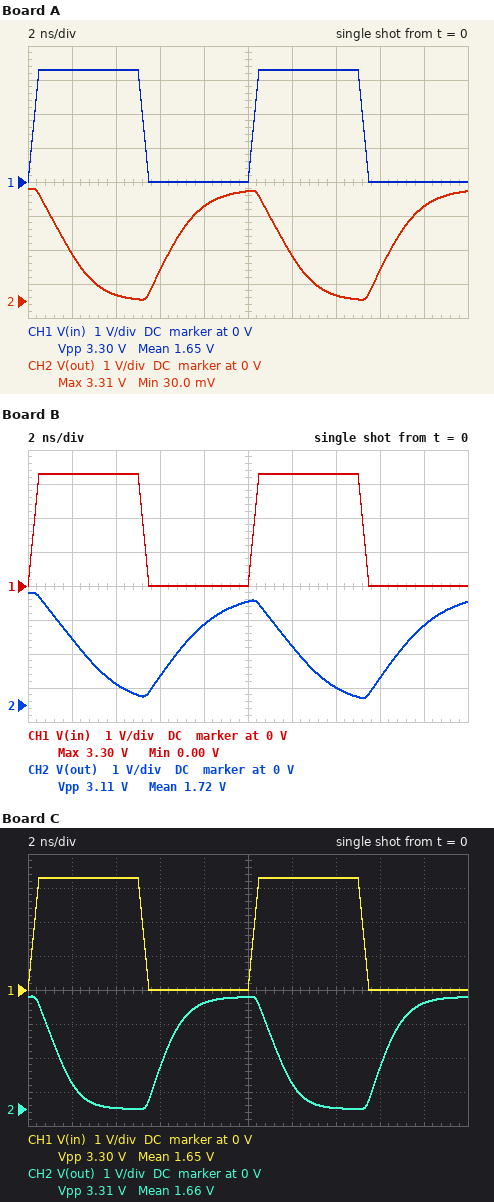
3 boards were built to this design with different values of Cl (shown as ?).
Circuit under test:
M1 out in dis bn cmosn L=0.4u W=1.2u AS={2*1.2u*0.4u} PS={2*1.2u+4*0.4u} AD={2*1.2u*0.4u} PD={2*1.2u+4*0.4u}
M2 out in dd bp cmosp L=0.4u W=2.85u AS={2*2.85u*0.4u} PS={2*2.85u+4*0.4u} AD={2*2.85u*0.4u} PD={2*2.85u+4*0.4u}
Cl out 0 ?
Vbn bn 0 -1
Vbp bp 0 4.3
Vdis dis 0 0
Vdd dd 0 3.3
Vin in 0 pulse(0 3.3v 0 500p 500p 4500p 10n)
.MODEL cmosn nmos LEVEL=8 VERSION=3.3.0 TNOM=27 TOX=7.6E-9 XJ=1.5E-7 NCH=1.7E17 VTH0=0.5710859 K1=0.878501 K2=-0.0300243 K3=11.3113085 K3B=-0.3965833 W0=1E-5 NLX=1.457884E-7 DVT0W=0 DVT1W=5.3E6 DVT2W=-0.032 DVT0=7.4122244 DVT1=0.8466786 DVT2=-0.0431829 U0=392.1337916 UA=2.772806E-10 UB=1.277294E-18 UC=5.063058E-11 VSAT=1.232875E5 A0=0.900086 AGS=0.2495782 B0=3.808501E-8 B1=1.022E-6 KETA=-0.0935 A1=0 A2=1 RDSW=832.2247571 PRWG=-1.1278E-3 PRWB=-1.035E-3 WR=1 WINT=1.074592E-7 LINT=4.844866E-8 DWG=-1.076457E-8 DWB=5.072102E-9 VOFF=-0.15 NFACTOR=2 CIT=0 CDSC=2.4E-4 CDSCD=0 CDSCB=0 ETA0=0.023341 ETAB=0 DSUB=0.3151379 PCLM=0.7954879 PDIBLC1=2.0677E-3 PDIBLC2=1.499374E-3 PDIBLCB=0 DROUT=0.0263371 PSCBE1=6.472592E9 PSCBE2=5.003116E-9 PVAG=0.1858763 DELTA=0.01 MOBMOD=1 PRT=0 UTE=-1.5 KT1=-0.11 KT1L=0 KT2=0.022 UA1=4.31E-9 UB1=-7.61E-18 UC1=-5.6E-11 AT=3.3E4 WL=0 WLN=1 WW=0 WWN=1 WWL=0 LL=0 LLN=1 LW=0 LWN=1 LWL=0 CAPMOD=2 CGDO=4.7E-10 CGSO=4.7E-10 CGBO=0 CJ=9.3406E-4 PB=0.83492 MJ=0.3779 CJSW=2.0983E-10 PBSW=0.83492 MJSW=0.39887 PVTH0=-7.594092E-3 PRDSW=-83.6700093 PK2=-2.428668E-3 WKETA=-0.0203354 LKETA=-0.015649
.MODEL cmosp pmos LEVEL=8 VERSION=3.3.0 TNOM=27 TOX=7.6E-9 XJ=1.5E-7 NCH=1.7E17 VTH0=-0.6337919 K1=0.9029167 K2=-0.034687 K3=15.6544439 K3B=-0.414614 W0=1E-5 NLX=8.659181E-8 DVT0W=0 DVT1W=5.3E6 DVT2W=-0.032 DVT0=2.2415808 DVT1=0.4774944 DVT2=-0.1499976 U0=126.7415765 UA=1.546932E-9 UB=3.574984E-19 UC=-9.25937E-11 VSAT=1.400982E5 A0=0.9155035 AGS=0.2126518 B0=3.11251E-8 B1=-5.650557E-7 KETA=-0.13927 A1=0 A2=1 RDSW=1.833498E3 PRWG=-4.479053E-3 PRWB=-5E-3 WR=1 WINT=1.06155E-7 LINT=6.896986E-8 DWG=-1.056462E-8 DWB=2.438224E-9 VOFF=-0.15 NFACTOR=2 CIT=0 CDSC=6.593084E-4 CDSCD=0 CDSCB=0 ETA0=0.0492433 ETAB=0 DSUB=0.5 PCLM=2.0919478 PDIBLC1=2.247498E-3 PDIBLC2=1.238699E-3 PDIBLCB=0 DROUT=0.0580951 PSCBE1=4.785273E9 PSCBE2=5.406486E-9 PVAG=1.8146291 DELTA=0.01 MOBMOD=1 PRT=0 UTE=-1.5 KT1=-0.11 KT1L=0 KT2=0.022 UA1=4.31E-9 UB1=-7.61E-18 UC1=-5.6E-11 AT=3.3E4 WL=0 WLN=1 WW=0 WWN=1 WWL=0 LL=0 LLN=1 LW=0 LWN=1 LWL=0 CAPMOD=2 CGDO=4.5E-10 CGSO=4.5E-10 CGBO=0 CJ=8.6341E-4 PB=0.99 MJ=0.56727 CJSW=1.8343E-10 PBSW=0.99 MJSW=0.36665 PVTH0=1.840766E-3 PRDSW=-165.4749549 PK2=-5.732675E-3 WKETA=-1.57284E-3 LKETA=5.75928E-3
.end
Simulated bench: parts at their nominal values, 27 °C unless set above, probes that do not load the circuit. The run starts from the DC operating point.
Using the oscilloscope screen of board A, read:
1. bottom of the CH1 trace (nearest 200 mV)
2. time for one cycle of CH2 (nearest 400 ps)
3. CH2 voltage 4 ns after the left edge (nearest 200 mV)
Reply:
0 V
10.0 ns
200 mV
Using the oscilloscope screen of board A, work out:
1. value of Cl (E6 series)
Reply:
470 fF
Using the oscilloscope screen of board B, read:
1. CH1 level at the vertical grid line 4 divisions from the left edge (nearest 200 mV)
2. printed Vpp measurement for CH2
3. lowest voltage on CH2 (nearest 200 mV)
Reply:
0 V
3.11 V
200 mV
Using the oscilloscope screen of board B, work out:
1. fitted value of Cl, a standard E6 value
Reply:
680 fF
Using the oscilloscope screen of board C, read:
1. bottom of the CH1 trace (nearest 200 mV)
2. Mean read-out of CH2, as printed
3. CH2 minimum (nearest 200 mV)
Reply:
0 V
1.66 V
0 V
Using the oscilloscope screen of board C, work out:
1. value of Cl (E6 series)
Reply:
330 fF
